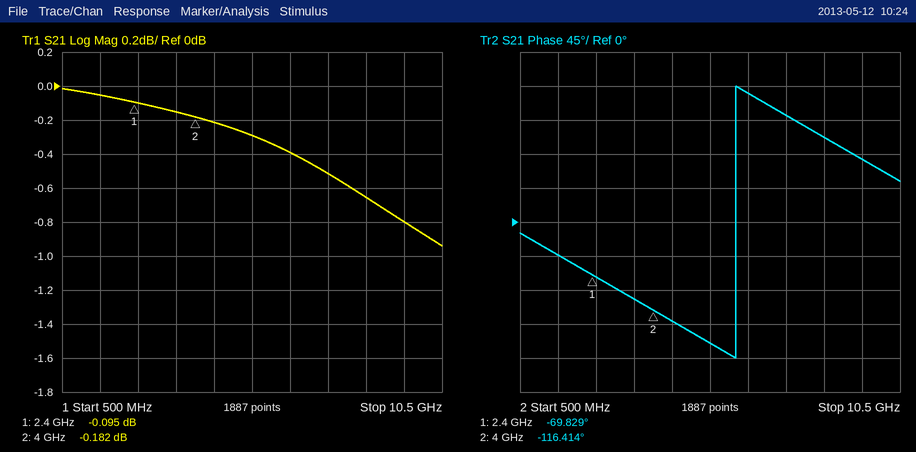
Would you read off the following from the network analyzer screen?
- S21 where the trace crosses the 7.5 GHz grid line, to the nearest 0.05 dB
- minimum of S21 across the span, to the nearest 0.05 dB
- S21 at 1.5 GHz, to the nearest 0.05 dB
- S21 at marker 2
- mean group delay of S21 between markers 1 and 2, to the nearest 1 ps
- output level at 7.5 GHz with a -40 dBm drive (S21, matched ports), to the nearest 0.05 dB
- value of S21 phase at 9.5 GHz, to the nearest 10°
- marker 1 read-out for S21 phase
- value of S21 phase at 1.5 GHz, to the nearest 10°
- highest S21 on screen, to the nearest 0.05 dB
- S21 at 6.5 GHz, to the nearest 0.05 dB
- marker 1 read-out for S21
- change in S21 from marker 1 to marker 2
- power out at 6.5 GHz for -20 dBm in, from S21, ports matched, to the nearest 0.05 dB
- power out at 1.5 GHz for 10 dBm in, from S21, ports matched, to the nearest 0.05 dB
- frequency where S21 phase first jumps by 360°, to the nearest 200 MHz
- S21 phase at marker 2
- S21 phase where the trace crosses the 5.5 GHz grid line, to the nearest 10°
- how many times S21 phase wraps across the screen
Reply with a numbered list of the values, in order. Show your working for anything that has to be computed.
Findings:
1. -0.50 dB
2. -0.95 dB
3. -0.05 dB
4. -0.182 dB
5. −(-116.414° − (-69.829°))/(360° × 1.6 GHz) ≈ 81 ps
6. -40 dBm + (-0.50 dB) = -40.50 dBm
7. 80°
8. -69.829°
9. -40°
10. 0.00 dB
11. -0.40 dB
12. -0.095 dB
13. -0.182 − (-0.095) = -0.087 dB
14. -20 dBm + (-0.40 dB) = -20.40 dBm
15. 10 dBm + (-0.05 dB) = 9.95 dBm
16. 6.2 GHz
17. -116.414°
18. -160°
19. 1
